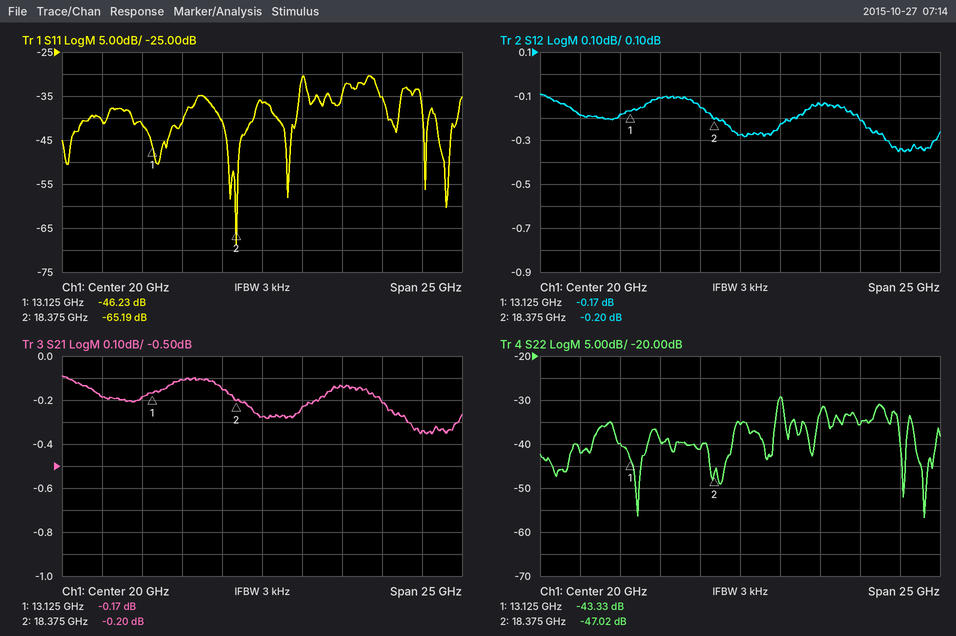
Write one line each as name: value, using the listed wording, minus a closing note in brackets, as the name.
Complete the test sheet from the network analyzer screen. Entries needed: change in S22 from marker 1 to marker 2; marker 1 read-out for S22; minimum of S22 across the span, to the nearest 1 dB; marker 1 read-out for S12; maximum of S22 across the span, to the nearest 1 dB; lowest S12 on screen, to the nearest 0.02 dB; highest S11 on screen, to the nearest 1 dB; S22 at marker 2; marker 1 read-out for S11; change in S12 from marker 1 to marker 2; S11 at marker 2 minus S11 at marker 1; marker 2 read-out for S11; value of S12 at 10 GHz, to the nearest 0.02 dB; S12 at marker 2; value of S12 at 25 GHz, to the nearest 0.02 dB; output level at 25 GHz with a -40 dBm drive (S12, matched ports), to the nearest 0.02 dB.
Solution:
change in S22 from marker 1 to marker 2: -3.69 dB
marker 1 read-out for S22: -43.33 dB
minimum of S22 across the span, to the nearest 1 dB: -57 dB
marker 1 read-out for S12: -0.17 dB
maximum of S22 across the span, to the nearest 1 dB: -29 dB
lowest S12 on screen, to the nearest 0.02 dB: -0.36 dB
highest S11 on screen, to the nearest 1 dB: -30 dB
S22 at marker 2: -47.02 dB
marker 1 read-out for S11: -46.23 dB
change in S12 from marker 1 to marker 2: -0.03 dB
S11 at marker 2 minus S11 at marker 1: -18.96 dB
marker 2 read-out for S11: -65.19 dB
value of S12 at 10 GHz, to the nearest 0.02 dB: -0.18 dB
S12 at marker 2: -0.20 dB
value of S12 at 25 GHz, to the nearest 0.02 dB: -0.14 dB
output level at 25 GHz with a -40 dBm drive (S12, matched ports), to the nearest 0.02 dB: -40.14 dBm
